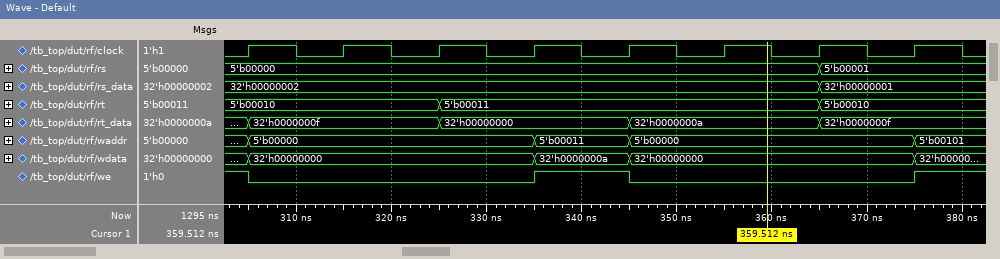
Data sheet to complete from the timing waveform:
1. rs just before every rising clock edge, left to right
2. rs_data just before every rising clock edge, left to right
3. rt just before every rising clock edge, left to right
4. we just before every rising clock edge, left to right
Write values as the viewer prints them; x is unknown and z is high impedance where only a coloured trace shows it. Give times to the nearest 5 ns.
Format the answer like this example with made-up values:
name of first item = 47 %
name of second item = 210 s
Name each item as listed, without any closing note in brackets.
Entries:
rs just before every rising clock edge, left to right = 5'b00000, 5'b00000, 5'b00000, 5'b00000, 5'b00000, 5'b00000, 5'b00000, 5'b00001
rs_data just before every rising clock edge, left to right = 32'h00000002, 32'h00000002, 32'h00000002, 32'h00000002, 32'h00000002, 32'h00000002, 32'h00000002, 32'h00000001
rt just before every rising clock edge, left to right = 5'b00010, 5'b00010, 5'b00010, 5'b00011, 5'b00011, 5'b00011, 5'b00011, 5'b00010
we just before every rising clock edge, left to right = 1 0 0 0 1 0 0 0
